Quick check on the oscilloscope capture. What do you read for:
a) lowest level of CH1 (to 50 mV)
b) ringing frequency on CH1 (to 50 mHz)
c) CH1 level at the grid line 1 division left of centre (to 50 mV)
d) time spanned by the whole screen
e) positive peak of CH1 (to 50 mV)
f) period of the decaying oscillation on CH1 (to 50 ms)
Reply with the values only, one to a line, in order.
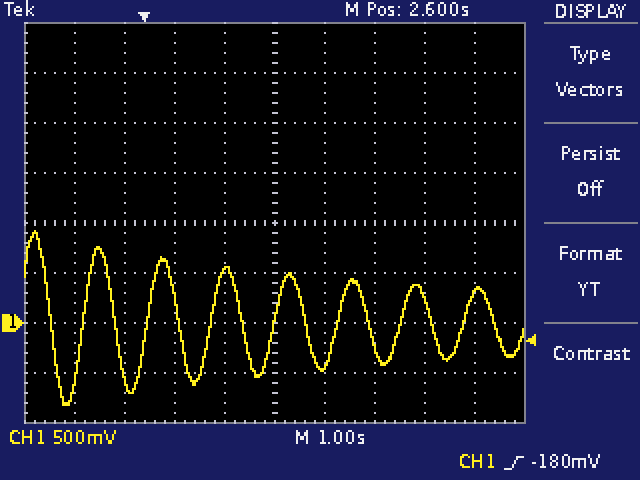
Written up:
-800 mV
800 mHz
500 mV
10 s
900 mV
1.25 s
